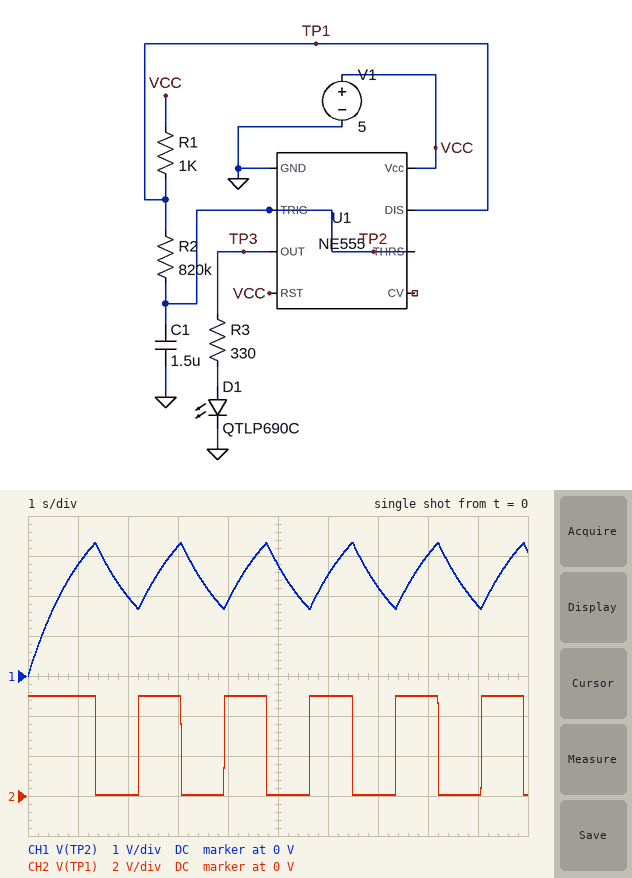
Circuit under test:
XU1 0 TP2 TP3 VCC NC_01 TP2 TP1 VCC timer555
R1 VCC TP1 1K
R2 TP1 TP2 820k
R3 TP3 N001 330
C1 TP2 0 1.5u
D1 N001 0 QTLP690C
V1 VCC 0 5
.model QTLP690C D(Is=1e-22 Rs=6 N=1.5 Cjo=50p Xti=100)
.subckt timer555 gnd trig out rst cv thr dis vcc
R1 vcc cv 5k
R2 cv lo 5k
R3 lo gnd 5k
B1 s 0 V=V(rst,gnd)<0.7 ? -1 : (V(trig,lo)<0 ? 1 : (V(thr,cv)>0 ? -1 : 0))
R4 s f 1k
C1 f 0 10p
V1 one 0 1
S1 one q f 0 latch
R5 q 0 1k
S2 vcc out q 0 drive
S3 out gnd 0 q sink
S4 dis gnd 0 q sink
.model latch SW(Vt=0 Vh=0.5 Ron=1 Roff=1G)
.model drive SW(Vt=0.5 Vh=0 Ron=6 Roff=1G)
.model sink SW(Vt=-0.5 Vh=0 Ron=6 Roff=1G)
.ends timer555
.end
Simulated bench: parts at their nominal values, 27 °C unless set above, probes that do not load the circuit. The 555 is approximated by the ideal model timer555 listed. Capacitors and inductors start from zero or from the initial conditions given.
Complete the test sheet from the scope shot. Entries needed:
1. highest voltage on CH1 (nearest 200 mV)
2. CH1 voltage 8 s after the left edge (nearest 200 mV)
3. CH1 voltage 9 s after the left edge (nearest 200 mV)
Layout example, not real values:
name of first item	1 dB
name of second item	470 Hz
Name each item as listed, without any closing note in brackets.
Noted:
highest voltage on CH1	3.4 V
CH1 voltage 8 s after the left edge	3.0 V
CH1 voltage 9 s after the left edge	1.8 V
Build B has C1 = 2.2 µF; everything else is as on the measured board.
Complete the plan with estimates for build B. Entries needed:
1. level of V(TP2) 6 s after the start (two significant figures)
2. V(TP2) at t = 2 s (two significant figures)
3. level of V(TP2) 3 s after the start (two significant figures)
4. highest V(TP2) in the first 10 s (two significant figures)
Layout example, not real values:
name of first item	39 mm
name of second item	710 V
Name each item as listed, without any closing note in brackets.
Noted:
level of V(TP2) 6 s after the start	2.1 V
V(TP2) at t = 2 s	3.3 V
level of V(TP2) 3 s after the start	1.9 V
highest V(TP2) in the first 10 s	3.3 V
